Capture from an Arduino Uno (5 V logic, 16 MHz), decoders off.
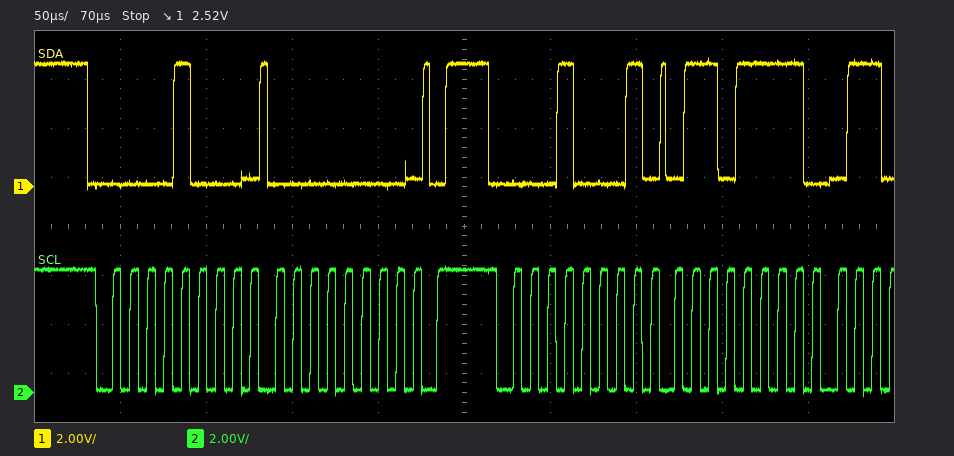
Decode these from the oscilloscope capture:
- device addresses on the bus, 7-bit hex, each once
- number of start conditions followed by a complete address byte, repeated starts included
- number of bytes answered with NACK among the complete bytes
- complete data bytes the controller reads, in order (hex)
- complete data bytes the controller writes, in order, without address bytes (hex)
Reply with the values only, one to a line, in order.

0x04 0x08
2
0
6F
00
